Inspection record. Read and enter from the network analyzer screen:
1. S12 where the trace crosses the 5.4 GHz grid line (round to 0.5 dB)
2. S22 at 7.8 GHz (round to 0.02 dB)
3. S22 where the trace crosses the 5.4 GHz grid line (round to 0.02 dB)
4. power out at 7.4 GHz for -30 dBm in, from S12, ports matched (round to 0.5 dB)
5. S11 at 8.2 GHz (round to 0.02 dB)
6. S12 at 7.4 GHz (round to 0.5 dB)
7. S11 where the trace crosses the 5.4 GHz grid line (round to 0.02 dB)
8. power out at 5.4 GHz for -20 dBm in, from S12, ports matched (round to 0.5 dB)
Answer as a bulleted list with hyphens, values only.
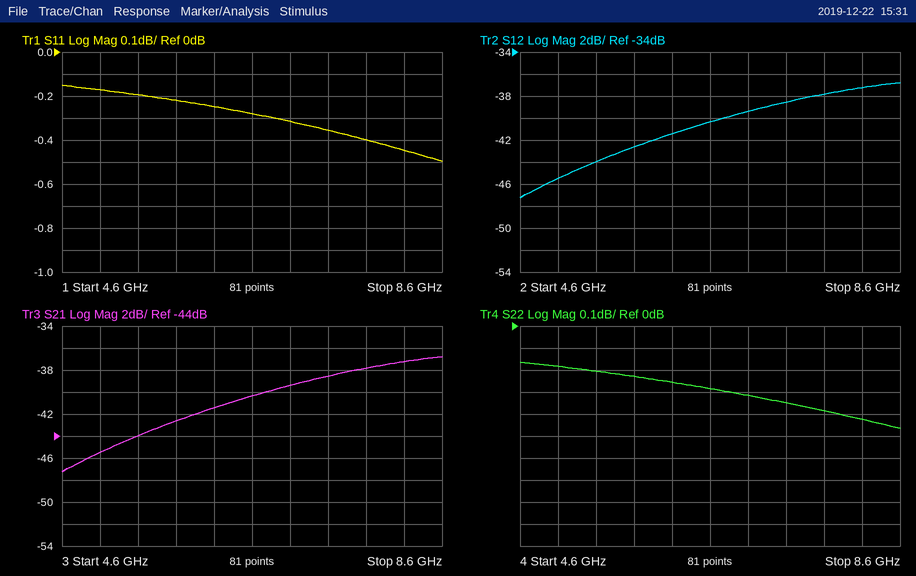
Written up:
- -44.0 dB
- -0.38 dB
- -0.20 dB
- -68.5 dBm
- -0.44 dB
- -38.5 dB
- -0.20 dB
- -64.0 dBm
